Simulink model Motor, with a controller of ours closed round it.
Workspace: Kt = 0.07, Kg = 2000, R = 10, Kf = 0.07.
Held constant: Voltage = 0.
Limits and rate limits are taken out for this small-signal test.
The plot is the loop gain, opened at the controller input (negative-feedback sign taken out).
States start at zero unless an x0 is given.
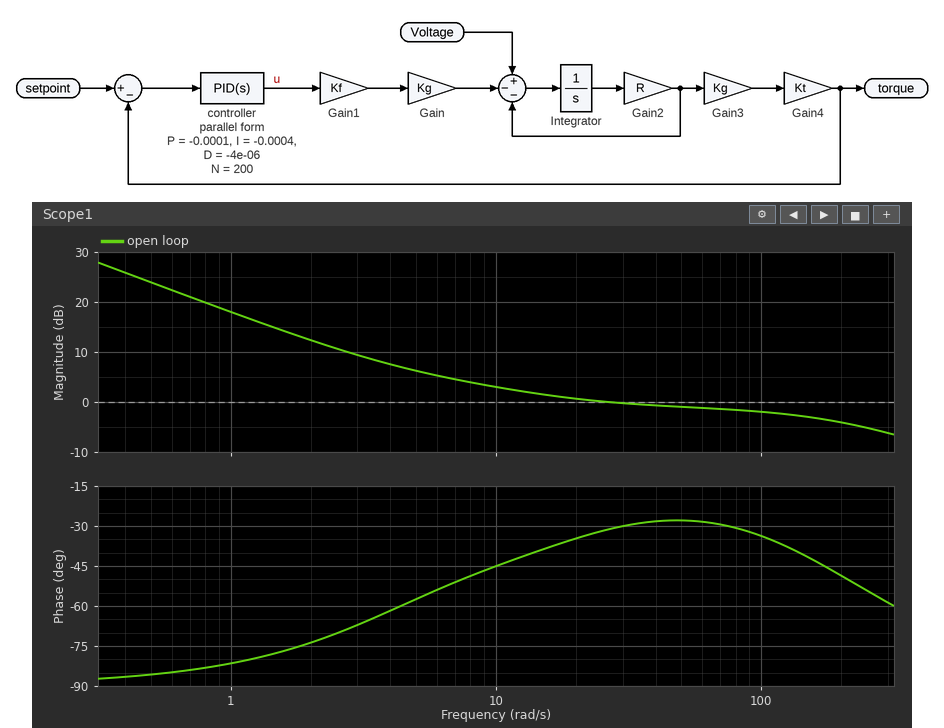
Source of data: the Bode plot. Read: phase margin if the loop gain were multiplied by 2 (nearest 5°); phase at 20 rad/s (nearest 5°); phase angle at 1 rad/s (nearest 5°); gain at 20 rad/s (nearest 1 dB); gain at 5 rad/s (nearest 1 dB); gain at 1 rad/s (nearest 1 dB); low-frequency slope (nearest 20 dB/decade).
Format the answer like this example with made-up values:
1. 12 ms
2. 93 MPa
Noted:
1. 120°
2. -35°
3. -80°
4. 1 dB
5. 6 dB
6. 18 dB
7. -20 dB/decade
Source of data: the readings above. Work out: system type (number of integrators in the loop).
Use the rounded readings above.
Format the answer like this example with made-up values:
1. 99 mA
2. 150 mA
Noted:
1. 1
